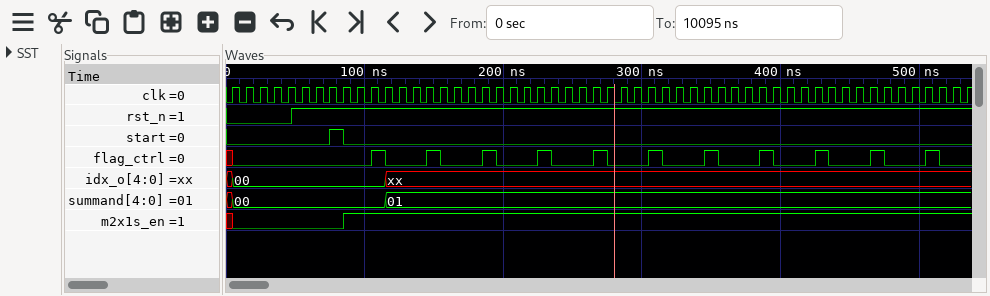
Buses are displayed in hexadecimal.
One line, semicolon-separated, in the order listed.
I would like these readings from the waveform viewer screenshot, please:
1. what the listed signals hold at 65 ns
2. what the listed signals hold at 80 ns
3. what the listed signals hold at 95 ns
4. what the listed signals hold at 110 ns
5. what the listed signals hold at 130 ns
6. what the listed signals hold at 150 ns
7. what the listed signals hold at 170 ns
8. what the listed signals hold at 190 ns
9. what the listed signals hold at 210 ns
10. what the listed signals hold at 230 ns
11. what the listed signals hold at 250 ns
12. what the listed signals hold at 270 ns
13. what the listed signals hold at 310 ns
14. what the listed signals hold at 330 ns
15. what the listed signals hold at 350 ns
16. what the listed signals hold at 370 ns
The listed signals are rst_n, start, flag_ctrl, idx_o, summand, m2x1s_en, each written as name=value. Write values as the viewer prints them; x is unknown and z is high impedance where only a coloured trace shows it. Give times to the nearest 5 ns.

rst_n=1, start=0, flag_ctrl=0, idx_o=00, summand=00, m2x1s_en=0; rst_n=1, start=1, flag_ctrl=0, idx_o=00, summand=00, m2x1s_en=0; rst_n=1, start=0, flag_ctrl=0, idx_o=00, summand=00, m2x1s_en=1; rst_n=1, start=0, flag_ctrl=1, idx_o=00, summand=00, m2x1s_en=1; rst_n=1, start=0, flag_ctrl=0, idx_o=xx, summand=01, m2x1s_en=1; rst_n=1, start=0, flag_ctrl=1, idx_o=xx, summand=01, m2x1s_en=1; rst_n=1, start=0, flag_ctrl=0, idx_o=xx, summand=01, m2x1s_en=1; rst_n=1, start=0, flag_ctrl=1, idx_o=xx, summand=01, m2x1s_en=1; rst_n=1, start=0, flag_ctrl=0, idx_o=xx, summand=01, m2x1s_en=1; rst_n=1, start=0, flag_ctrl=1, idx_o=xx, summand=01, m2x1s_en=1; rst_n=1, start=0, flag_ctrl=0, idx_o=xx, summand=01, m2x1s_en=1; rst_n=1, start=0, flag_ctrl=1, idx_o=xx, summand=01, m2x1s_en=1; rst_n=1, start=0, flag_ctrl=1, idx_o=xx, summand=01, m2x1s_en=1; rst_n=1, start=0, flag_ctrl=0, idx_o=xx, summand=01, m2x1s_en=1; rst_n=1, start=0, flag_ctrl=1, idx_o=xx, summand=01, m2x1s_en=1; rst_n=1, start=0, flag_ctrl=0, idx_o=xx, summand=01, m2x1s_en=1
